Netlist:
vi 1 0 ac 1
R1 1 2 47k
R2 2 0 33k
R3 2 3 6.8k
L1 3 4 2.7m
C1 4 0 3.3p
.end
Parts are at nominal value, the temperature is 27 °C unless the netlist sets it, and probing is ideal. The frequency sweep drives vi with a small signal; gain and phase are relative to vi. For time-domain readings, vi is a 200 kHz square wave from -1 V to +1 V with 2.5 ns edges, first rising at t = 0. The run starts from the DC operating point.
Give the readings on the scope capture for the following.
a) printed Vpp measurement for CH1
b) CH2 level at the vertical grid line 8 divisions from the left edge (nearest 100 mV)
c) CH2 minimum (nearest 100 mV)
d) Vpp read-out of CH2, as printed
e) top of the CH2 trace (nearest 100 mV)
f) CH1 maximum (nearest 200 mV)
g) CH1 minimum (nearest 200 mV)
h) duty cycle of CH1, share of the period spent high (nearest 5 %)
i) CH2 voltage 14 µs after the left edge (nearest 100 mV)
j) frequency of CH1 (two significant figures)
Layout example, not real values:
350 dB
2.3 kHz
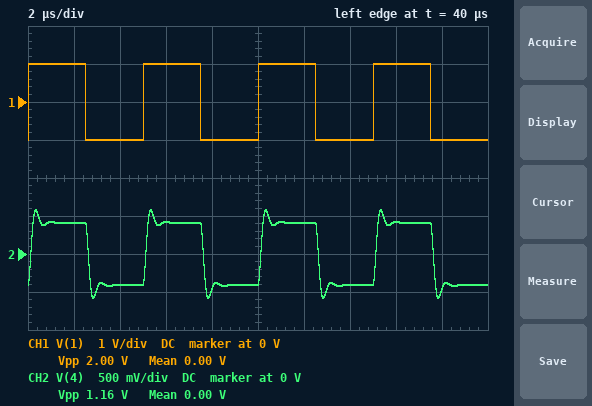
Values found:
2.00 V
400 mV
-600 mV
1.16 V
600 mV
1.0 V
-1.0 V
50 %
-400 mV
200 kHz
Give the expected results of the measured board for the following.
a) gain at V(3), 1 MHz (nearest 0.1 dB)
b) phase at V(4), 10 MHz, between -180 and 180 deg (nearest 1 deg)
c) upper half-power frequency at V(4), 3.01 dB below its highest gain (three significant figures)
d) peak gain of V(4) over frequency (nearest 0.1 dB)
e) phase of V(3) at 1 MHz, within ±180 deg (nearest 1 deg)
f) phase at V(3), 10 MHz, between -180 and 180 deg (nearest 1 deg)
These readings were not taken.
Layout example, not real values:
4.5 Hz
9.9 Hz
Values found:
-10.0 dB
-171 deg
1.99 MHz
-5.9 dB
-40 deg
9 deg
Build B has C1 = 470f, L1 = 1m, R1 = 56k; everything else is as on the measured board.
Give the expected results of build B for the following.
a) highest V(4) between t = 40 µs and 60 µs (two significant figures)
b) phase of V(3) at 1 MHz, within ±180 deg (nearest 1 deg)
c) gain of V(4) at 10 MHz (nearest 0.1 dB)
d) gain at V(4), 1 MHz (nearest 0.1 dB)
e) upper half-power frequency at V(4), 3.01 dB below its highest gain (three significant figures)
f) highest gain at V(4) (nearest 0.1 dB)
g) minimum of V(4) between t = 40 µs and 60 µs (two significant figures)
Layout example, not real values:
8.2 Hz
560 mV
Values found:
650 mV
-5 deg
-10.1 dB
-8.5 dB
8.66 MHz
-3.7 dB
-650 mV
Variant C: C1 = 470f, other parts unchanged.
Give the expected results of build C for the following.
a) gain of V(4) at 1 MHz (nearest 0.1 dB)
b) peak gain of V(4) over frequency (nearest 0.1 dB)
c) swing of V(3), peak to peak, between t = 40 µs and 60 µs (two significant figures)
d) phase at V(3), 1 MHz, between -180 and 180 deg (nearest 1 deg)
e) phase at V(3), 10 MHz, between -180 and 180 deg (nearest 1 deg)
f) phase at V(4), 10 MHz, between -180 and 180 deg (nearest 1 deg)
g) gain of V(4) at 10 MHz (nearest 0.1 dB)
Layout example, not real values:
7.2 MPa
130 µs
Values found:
-7.3 dB
1.7 dB
1.1 V
-5 deg
11 deg
-169 deg
-19.9 dB
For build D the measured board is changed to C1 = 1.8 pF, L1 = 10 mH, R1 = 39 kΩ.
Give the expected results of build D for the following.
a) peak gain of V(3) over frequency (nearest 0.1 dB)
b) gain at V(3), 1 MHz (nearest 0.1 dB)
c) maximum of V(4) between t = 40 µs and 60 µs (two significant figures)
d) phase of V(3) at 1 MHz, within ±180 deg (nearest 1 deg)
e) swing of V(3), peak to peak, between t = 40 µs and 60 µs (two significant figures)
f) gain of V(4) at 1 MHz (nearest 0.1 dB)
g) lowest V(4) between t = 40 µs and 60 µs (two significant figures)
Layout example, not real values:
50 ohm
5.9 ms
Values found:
-6.8 dB
-9.6 dB
980 mV
-44 deg
1.2 V
1.1 dB
-980 mV
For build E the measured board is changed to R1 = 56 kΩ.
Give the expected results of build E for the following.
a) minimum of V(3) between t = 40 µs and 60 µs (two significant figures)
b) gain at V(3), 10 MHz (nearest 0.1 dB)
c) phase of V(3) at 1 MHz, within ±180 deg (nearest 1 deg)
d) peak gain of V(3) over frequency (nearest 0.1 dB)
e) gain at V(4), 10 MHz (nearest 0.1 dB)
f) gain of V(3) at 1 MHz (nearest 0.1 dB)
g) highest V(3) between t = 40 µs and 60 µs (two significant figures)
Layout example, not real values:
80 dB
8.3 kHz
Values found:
-440 mV
-8.7 dB
-41 deg
-8.6 dB
-39.4 dB
-11.1 dB
440 mV
